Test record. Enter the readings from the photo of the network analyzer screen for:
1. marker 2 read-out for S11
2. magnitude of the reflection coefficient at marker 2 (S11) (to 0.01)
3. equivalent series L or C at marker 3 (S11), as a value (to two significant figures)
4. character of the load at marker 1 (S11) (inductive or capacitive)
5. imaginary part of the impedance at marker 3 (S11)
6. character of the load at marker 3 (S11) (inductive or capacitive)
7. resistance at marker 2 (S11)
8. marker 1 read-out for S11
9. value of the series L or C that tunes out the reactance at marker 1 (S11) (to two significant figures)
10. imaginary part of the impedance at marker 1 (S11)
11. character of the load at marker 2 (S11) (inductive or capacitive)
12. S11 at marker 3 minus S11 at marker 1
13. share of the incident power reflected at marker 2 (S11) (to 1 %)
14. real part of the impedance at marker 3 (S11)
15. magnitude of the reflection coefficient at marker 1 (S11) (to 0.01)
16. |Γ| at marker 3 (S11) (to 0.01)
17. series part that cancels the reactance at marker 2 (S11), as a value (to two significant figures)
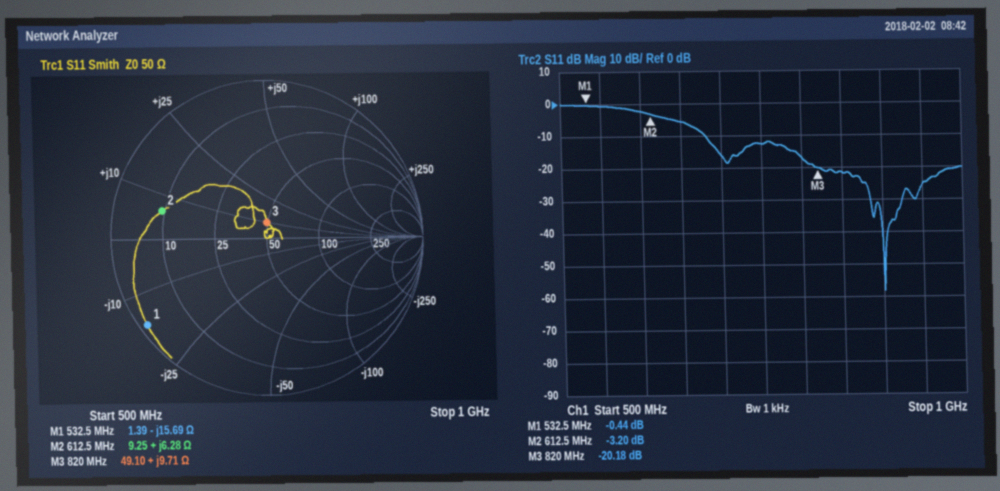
-3.20 dB
0.69
1.9 nH
capacitive
+9.71 Ω
inductive
9.25 Ω
-0.44 dB
4.7 nH
-15.69 Ω
inductive
-19.74 dB
48 %
49.10 Ω
0.95
0.10
41 pF
